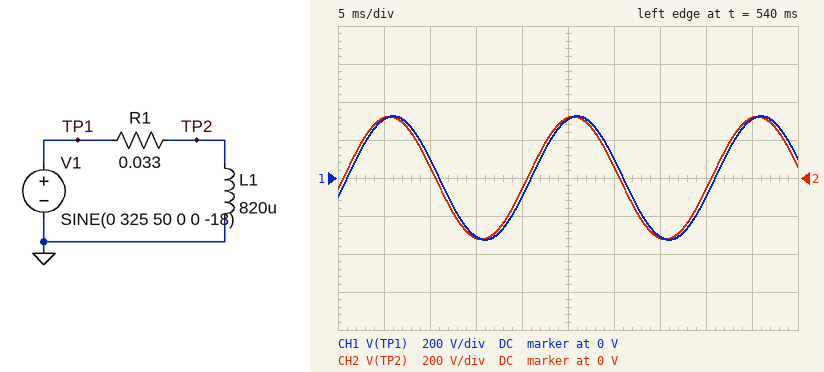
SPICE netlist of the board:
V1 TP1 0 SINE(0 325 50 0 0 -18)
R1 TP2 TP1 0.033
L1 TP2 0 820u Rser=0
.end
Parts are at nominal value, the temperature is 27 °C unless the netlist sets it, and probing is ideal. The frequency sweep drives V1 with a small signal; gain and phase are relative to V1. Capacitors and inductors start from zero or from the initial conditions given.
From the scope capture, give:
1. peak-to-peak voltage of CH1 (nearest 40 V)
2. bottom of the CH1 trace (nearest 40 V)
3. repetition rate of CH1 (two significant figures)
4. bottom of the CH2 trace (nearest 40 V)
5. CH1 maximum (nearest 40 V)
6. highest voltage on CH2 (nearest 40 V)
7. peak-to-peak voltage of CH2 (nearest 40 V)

640 V
-320 V
50 Hz
-320 V
320 V
320 V
640 V
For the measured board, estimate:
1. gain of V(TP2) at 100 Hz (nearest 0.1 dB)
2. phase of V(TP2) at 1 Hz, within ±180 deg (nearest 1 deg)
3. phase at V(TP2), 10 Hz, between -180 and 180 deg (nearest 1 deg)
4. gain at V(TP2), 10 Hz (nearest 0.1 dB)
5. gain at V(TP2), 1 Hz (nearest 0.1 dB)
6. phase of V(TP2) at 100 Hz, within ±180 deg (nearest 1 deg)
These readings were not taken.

0 dB
81 deg
33 deg
-1.5 dB
-16.2 dB
4 deg
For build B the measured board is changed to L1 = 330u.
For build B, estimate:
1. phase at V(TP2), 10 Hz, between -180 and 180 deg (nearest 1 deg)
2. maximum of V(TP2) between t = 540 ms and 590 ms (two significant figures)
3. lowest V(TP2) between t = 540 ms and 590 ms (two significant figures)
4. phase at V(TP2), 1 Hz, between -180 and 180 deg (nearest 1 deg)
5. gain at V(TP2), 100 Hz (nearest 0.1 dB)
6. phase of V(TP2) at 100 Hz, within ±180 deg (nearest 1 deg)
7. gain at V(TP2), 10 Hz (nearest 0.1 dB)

58 deg
310 V
-310 V
86 deg
-0.1 dB
9 deg
-5.5 dB
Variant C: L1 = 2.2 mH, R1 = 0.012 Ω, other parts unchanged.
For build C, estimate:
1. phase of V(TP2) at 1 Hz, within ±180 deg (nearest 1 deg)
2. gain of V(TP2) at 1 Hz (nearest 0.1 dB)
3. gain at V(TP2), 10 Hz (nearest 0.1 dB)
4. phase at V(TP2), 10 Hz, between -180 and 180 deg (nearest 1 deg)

41 deg
-2.4 dB
0 dB
5 deg
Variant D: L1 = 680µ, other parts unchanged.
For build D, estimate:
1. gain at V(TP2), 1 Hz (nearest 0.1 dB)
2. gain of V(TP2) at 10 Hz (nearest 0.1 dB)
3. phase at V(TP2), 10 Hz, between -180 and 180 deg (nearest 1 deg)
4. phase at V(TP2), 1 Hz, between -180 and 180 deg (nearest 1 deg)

-17.8 dB
-2.0 dB
38 deg
83 deg
